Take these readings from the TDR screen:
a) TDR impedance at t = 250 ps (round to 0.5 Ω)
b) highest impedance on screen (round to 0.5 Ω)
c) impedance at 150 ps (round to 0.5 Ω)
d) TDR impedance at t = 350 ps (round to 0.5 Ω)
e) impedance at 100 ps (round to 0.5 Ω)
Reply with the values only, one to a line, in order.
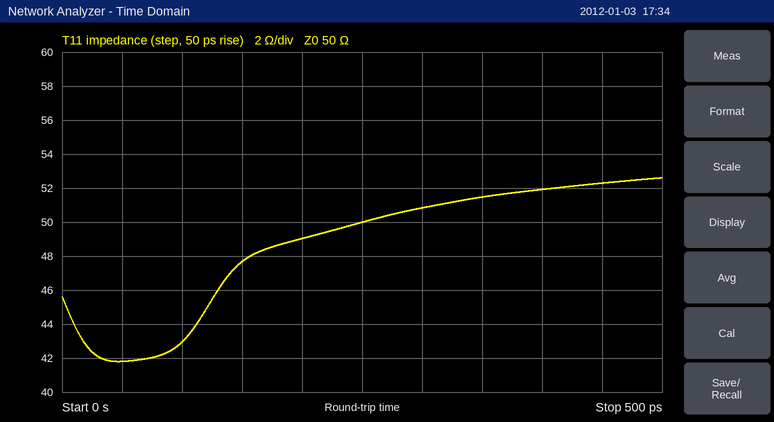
50.0 Ω
52.5 Ω
47.5 Ω
51.5 Ω
43.0 Ω
